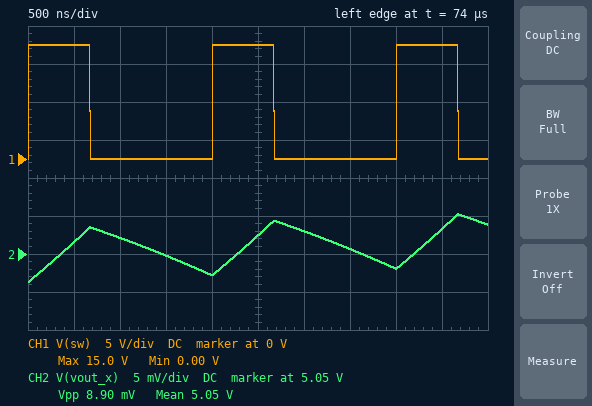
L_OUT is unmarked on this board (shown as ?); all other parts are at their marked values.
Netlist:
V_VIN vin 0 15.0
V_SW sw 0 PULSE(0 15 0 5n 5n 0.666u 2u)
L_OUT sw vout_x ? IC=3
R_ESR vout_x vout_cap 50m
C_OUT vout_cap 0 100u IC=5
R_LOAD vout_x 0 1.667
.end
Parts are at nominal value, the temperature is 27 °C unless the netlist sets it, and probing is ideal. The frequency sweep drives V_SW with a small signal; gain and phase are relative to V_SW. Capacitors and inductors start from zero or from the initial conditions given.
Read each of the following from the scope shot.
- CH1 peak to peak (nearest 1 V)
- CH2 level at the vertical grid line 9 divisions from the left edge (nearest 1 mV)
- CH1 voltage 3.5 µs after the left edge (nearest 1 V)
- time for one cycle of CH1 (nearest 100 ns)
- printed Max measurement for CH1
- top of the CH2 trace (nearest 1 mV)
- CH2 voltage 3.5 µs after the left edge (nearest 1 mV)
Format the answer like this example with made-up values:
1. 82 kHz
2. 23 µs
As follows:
1. 15 V
2. 5.053 V
3. 0 V
4. 2.0 µs
5. 15.0 V
6. 5.055 V
7. 5.051 V
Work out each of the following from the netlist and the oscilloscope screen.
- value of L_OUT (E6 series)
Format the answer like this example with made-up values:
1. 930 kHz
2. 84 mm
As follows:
1. 47 µH
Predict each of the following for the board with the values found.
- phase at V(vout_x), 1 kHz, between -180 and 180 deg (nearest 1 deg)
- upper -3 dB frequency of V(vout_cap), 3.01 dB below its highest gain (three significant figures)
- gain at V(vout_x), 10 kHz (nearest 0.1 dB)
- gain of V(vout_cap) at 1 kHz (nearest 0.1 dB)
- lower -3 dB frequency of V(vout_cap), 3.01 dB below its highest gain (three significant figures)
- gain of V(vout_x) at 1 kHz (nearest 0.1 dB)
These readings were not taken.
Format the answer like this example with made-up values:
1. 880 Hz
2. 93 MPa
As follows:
1. -13 deg
2. 2.66 kHz
3. -24.8 dB
4. 1.6 dB
5. 1.49 kHz
6. 1.6 dB
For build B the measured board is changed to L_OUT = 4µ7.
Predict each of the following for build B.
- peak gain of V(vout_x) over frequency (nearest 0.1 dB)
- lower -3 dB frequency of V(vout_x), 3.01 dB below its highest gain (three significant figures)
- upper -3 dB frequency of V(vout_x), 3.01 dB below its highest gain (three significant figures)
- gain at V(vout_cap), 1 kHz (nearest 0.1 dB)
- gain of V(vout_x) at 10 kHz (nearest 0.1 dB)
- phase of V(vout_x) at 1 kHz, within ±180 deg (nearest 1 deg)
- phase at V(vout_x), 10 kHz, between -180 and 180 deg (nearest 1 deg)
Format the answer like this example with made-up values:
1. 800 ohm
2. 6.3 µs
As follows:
1. 9.3 dB
2. 5.57 kHz
3. 8.22 kHz
4. 0.2 dB
5. 0.1 dB
6. -1 deg
7. -134 deg
